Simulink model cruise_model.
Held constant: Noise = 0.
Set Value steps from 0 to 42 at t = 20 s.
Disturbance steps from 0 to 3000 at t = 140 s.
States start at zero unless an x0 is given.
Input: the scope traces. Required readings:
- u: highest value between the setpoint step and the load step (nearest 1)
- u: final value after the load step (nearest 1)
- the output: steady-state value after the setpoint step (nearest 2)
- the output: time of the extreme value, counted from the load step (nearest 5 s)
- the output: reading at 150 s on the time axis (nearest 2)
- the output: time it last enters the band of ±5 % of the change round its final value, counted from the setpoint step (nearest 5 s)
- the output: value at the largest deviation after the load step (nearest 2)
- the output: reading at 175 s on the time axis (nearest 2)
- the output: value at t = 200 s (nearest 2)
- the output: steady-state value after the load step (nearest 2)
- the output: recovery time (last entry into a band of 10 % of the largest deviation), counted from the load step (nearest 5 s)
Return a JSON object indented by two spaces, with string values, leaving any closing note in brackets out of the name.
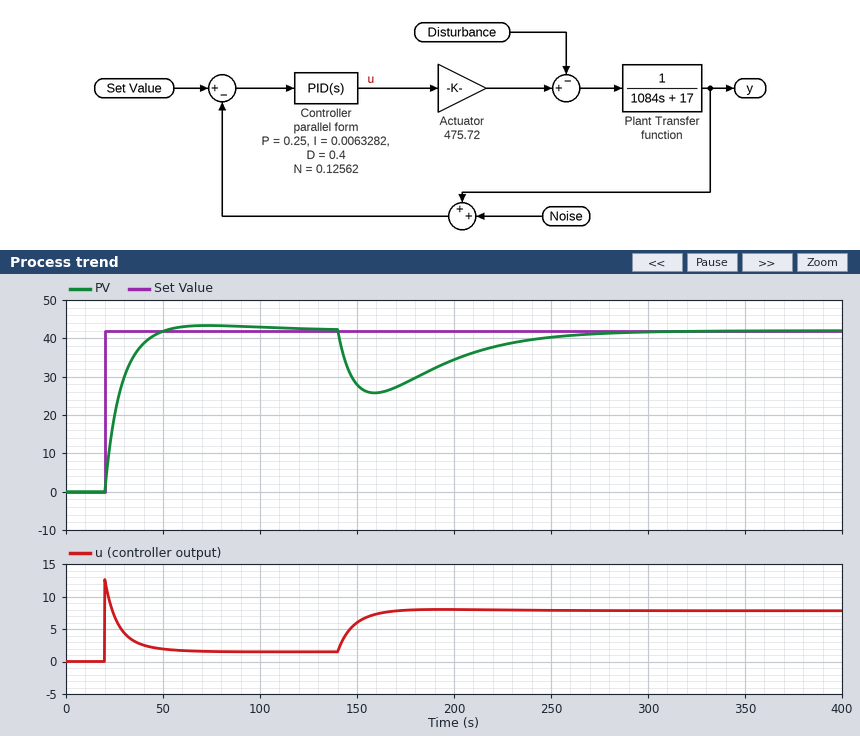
{
  "u: highest value between the setpoint step and the load step": "13",
  "u: final value after the load step": "8",
  "the output: steady-state value after the setpoint step": "42",
  "the output: time of the extreme value, counted from the load step": "20 s",
  "the output: reading at 150 s on the time axis": "28",
  "the output: time it last enters the band of ±5 % of the change round its final value, counted from the setpoint step": "25 s",
  "the output: value at the largest deviation after the load step": "26",
  "the output: reading at 175 s on the time axis": "28",
  "the output: value at t = 200 s": "34",
  "the output: steady-state value after the load step": "42",
  "the output: recovery time (last entry into a band of 10 % of the largest deviation), counted from the load step": "110 s"
}
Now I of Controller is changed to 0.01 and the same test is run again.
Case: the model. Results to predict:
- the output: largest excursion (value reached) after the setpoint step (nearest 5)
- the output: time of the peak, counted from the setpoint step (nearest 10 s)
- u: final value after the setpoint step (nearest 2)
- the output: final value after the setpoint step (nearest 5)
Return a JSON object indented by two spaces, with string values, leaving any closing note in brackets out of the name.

{
  "the output: largest excursion (value reached) after the setpoint step": "45",
  "the output: time of the peak, counted from the setpoint step": "40 s",
  "u: final value after the setpoint step": "2",
  "the output: final value after the setpoint step": "40"
}
